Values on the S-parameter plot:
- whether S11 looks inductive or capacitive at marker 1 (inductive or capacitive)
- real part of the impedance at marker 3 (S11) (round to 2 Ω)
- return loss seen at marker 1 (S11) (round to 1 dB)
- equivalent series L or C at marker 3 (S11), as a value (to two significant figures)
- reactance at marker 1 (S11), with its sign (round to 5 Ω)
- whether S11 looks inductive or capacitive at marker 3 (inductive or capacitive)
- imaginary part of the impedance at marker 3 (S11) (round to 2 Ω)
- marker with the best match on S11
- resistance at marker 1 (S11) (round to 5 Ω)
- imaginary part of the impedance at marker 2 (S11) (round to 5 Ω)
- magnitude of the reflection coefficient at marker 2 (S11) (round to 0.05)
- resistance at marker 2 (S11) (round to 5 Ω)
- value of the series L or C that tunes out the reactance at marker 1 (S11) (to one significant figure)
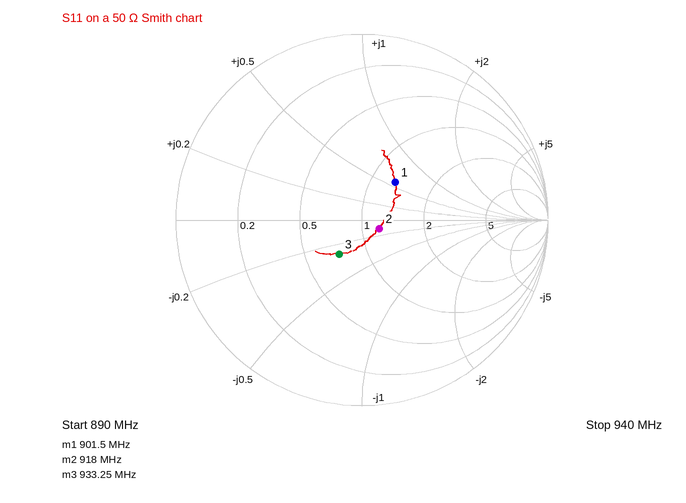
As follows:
inductive
36 Ω
11 dB
12 pF
+30 Ω
capacitive
-14 Ω
marker 2
65 Ω
-5 Ω
0.10
60 Ω
6 pF
